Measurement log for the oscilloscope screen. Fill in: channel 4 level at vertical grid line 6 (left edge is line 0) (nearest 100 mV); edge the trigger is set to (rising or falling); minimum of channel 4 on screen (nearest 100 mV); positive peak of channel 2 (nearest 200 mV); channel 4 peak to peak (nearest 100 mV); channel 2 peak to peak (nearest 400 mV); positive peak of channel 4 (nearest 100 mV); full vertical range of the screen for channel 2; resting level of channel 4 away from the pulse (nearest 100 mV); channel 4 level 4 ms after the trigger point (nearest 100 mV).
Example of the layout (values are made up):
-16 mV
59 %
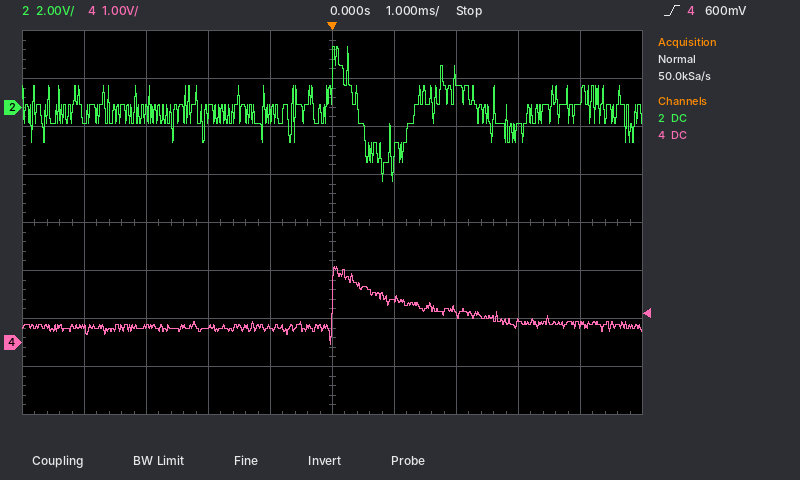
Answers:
900 mV
rising
0.0 V
2.6 V
1.6 V
5.6 V
1.6 V
16 V
300 mV
400 mV
